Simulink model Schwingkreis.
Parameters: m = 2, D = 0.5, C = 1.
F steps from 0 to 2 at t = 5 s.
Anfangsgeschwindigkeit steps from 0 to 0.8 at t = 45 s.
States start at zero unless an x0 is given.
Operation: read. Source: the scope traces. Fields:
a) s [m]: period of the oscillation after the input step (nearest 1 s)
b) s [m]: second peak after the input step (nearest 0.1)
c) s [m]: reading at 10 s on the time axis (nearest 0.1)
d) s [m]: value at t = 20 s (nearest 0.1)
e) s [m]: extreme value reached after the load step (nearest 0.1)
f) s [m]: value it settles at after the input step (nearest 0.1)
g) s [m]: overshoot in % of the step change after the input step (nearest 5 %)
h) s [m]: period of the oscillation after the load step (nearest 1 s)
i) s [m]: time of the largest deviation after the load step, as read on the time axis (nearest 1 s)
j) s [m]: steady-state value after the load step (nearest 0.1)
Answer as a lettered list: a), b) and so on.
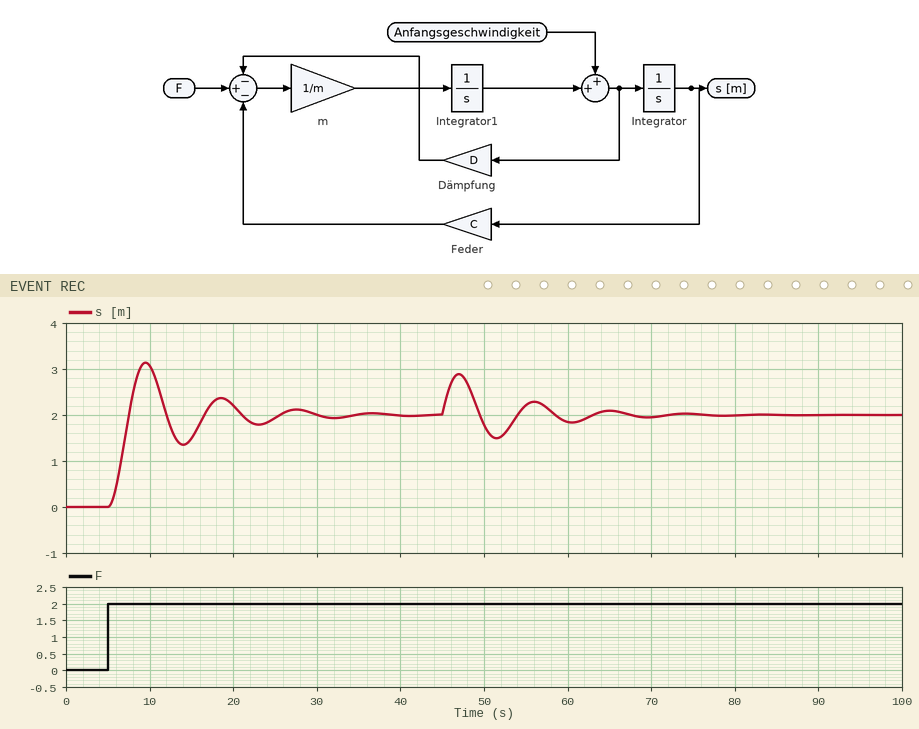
a) 9 s
b) 2.4
c) 3.1
d) 2.2
e) 2.9
f) 2.0
g) 55 %
h) 9 s
i) 47 s
j) 2.0
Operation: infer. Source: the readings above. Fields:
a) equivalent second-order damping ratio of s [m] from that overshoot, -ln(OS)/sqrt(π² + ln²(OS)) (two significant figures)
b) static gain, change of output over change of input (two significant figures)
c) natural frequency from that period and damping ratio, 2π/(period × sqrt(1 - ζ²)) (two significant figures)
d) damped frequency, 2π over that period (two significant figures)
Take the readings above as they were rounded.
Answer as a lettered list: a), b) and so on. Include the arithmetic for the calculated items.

a) ln(0.55) = -0.598; 0.598 / sqrt(9.870 + 0.357) = 0.19
b) (2 - 0) / (2 - 0) = 1.0
c) 2π / (9 × sqrt(1 - 0.19²)) = 0.71 rad/s
d) 2π / 9 = 0.70 rad/s
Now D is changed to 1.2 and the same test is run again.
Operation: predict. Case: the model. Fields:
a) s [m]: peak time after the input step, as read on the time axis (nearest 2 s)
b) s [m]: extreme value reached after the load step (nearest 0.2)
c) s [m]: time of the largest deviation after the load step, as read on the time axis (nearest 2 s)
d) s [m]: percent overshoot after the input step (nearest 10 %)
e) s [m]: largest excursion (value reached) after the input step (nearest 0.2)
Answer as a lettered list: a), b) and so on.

a) 10 s
b) 2.6
c) 46 s
d) 20 %
e) 2.4
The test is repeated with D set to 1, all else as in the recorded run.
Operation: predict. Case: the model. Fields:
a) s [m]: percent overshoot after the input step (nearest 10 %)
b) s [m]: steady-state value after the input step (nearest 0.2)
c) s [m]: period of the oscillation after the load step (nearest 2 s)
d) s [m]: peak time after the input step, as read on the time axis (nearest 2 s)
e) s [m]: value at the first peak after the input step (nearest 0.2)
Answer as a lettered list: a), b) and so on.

a) 30 %
b) 2.0
c) 10 s
d) 10 s
e) 2.6
